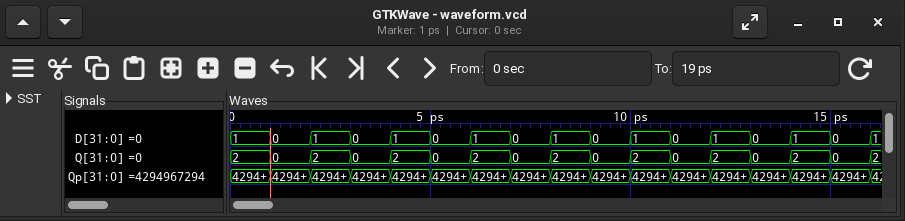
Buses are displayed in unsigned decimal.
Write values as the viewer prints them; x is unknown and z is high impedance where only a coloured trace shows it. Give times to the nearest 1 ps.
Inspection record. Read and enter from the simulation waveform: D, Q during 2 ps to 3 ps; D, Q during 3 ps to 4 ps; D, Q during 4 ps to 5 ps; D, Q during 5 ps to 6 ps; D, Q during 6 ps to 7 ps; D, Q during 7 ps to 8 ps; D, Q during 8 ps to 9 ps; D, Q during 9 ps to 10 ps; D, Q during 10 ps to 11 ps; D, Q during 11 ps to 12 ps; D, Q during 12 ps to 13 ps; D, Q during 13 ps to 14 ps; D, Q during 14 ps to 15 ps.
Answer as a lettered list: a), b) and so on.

a) D=1, Q=2
b) D=0, Q=0
c) D=1, Q=2
d) D=0, Q=0
e) D=1, Q=2
f) D=0, Q=0
g) D=1, Q=2
h) D=0, Q=0
i) D=1, Q=2
j) D=0, Q=0
k) D=1, Q=2
l) D=0, Q=0
m) D=1, Q=2
